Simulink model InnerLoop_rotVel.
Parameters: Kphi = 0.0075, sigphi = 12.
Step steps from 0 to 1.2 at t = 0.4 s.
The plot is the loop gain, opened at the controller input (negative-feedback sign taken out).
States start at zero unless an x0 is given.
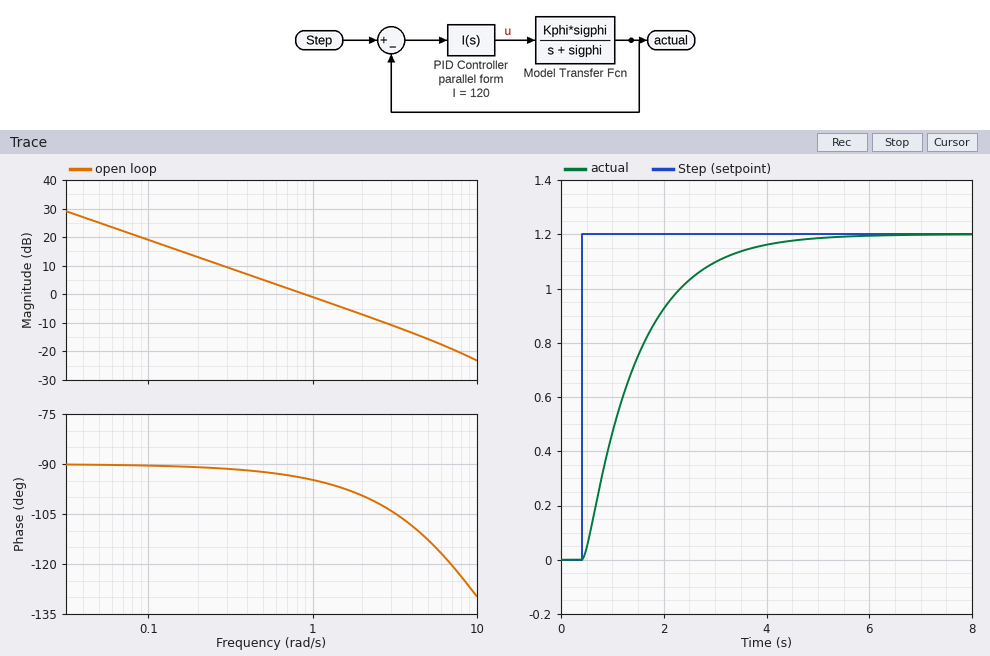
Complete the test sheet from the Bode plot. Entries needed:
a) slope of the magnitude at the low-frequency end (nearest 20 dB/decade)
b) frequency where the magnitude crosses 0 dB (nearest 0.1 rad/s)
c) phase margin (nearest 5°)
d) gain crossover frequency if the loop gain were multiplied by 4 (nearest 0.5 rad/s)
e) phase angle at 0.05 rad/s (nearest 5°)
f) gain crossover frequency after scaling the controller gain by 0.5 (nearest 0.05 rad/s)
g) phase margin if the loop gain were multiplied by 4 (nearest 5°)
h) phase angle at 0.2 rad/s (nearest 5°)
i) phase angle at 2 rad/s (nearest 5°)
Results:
-20 dB/decade
0.9 rad/s
85°
3.5 rad/s
-90°
0.45 rad/s
75°
-90°
-100°
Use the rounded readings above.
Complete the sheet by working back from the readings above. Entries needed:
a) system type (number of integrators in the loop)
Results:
1
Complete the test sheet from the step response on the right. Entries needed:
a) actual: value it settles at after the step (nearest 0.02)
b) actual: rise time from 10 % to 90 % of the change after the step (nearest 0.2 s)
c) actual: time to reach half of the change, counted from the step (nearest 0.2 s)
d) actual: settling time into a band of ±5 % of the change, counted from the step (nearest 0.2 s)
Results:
1.20
2.2 s
0.8 s
3.2 s
